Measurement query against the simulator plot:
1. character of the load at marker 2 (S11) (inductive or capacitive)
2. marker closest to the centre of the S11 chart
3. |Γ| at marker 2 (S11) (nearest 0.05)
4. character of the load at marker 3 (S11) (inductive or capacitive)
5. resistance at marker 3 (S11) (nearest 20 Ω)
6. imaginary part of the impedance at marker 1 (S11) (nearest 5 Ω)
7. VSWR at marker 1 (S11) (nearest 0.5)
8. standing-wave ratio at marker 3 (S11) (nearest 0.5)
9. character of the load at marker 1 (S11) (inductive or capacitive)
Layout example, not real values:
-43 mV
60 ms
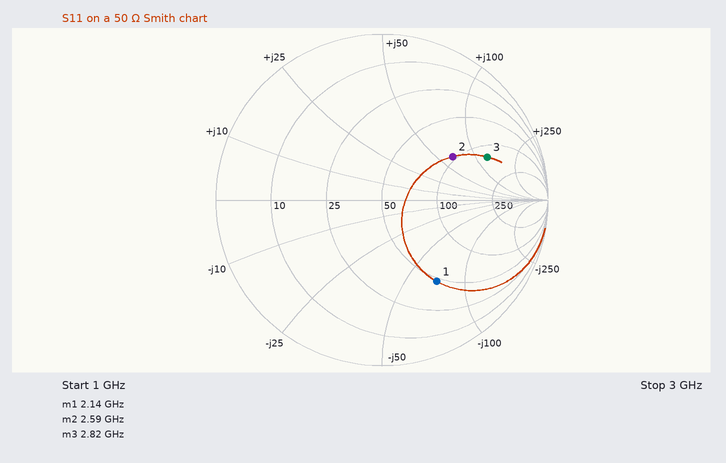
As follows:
inductive
marker 2
0.50
inductive
140 Ω
-70 Ω
4.0
5.5
capacitive
